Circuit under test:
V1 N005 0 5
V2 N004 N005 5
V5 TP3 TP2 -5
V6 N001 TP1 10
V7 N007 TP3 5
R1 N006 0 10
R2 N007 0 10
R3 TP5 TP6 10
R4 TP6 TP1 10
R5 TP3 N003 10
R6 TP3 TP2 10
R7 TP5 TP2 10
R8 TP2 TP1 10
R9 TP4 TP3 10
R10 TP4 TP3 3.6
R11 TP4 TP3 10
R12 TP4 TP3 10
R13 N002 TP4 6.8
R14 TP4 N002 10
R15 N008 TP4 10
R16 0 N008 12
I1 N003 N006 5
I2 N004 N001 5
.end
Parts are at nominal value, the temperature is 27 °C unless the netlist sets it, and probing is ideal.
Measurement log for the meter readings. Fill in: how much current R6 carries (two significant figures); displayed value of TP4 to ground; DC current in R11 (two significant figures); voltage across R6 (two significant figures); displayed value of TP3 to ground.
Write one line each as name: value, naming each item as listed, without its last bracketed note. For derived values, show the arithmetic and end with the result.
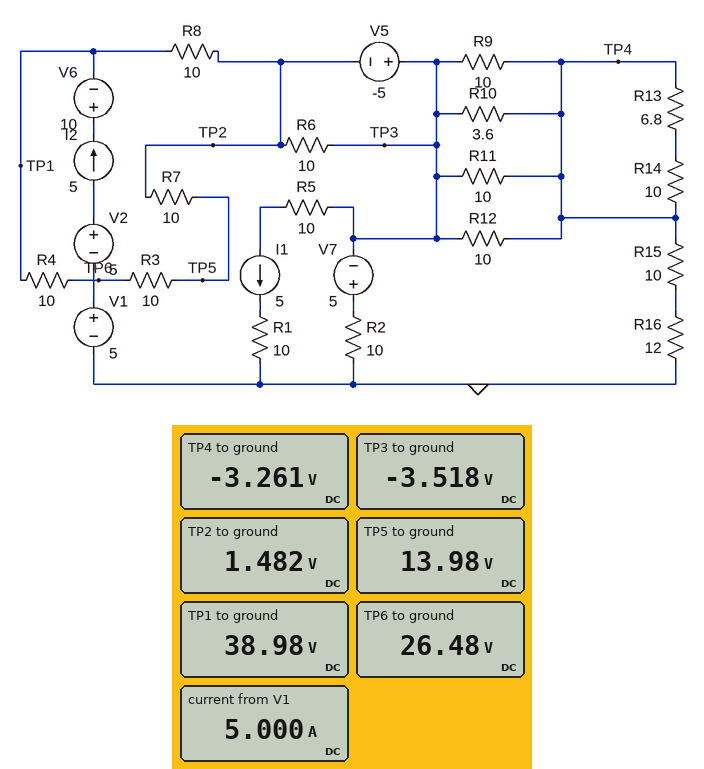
how much current R6 carries: (1.482 V - (-3.518 V)) / 10 Ω = 500 mA
displayed value of TP4 to ground: -3.261 V
DC current in R11: (-3.261 V - (-3.518 V)) / 10 Ω = 26 mA
voltage across R6: 1.482 V - (-3.518 V) = 5.0 V
displayed value of TP3 to ground: -3.518 V
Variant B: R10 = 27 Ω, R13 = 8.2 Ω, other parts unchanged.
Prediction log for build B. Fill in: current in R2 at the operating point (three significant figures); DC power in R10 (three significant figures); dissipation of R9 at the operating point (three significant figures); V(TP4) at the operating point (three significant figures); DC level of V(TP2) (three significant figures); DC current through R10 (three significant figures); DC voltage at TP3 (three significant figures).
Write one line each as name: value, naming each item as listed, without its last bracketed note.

current in R2 at the operating point: 143 mA
DC power in R10: 6.67 mW
dissipation of R9 at the operating point: 18.0 mW
V(TP4) at the operating point: -3.15 V
DC level of V(TP2): 1.43 V
DC current through R10: 15.7 mA
DC voltage at TP3: -3.57 V
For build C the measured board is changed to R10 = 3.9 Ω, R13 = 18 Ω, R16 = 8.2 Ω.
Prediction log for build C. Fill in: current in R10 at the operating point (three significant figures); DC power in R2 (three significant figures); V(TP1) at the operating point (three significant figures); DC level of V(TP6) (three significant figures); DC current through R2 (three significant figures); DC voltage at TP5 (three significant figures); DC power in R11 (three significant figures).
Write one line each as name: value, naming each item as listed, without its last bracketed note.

current in R10 at the operating point: 76.8 mA
DC power in R2: 278 mW
V(TP1) at the operating point: 39.2 V
DC level of V(TP6): 26.7 V
DC current through R2: 167 mA
DC voltage at TP5: 14.2 V
DC power in R11: 8.97 mW
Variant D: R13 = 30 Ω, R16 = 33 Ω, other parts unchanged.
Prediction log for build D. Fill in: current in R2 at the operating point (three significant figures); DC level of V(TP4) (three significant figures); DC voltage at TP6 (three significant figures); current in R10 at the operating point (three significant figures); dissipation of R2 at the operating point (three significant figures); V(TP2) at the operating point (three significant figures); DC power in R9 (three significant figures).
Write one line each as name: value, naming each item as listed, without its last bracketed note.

current in R2 at the operating point: 91.4 mA
DC level of V(TP4): -3.93 V
DC voltage at TP6: 25.9 V
current in R10 at the operating point: 43.9 mA
dissipation of R2 at the operating point: 83.5 mW
V(TP2) at the operating point: 914 mV
DC power in R9: 2.50 mW
